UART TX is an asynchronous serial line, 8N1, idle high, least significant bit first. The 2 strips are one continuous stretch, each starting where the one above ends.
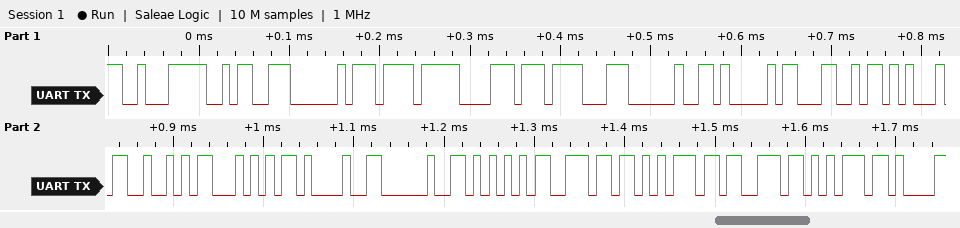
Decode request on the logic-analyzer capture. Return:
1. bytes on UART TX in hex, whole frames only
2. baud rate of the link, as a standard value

E2 9A A0 EF B8 8F 20 41 4C 45 52 54 21 20 55 6E 75 73 75
115200 baud
